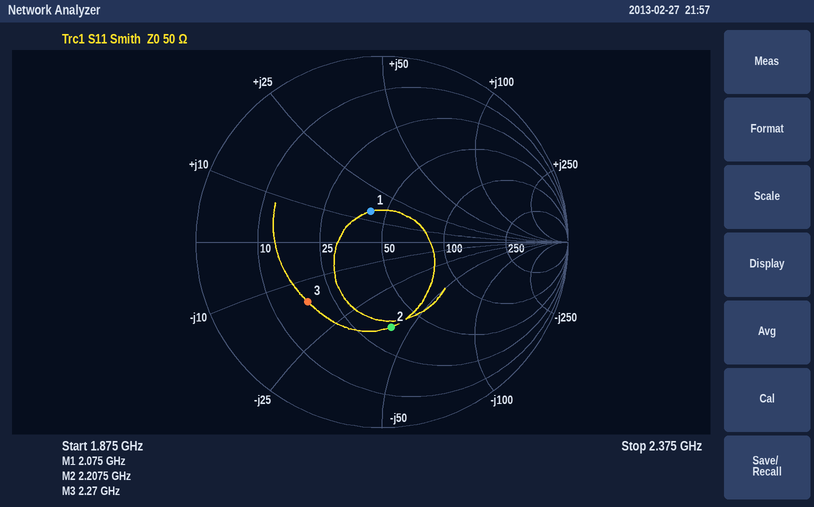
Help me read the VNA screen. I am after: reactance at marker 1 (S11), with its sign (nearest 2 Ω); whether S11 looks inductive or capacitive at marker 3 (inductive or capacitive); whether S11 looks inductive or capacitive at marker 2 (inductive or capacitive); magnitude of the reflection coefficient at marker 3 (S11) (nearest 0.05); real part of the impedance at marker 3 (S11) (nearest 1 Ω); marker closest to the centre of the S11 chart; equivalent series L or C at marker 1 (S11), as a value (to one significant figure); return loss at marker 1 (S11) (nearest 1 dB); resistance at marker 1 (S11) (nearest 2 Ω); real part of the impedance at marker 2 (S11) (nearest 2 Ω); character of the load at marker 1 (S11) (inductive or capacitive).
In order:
+14 Ω
capacitive
capacitive
0.50
18 Ω
marker 1
1 nH
15 dB
42 Ω
36 Ω
inductive
